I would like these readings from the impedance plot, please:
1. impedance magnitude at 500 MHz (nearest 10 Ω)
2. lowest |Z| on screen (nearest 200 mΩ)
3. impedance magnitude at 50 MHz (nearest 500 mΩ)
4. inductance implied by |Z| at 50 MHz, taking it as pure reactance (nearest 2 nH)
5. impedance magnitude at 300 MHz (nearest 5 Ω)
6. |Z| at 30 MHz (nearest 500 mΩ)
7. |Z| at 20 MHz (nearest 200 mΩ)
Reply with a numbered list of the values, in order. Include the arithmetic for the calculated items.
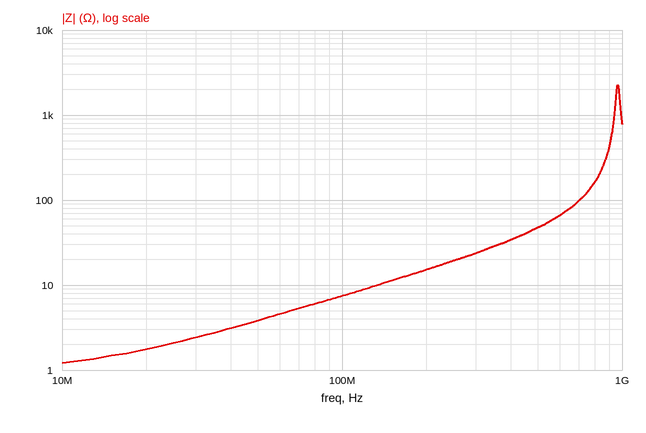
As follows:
1. 50 Ω
2. 1.2 Ω
3. 4.0 Ω
4. L = 4.0 Ω/(2π × 50 MHz) ≈ 12.7 nH, so 12 nH to the nearest 2 nH
5. 25 Ω
6. 2.5 Ω
7. 1.8 Ω
